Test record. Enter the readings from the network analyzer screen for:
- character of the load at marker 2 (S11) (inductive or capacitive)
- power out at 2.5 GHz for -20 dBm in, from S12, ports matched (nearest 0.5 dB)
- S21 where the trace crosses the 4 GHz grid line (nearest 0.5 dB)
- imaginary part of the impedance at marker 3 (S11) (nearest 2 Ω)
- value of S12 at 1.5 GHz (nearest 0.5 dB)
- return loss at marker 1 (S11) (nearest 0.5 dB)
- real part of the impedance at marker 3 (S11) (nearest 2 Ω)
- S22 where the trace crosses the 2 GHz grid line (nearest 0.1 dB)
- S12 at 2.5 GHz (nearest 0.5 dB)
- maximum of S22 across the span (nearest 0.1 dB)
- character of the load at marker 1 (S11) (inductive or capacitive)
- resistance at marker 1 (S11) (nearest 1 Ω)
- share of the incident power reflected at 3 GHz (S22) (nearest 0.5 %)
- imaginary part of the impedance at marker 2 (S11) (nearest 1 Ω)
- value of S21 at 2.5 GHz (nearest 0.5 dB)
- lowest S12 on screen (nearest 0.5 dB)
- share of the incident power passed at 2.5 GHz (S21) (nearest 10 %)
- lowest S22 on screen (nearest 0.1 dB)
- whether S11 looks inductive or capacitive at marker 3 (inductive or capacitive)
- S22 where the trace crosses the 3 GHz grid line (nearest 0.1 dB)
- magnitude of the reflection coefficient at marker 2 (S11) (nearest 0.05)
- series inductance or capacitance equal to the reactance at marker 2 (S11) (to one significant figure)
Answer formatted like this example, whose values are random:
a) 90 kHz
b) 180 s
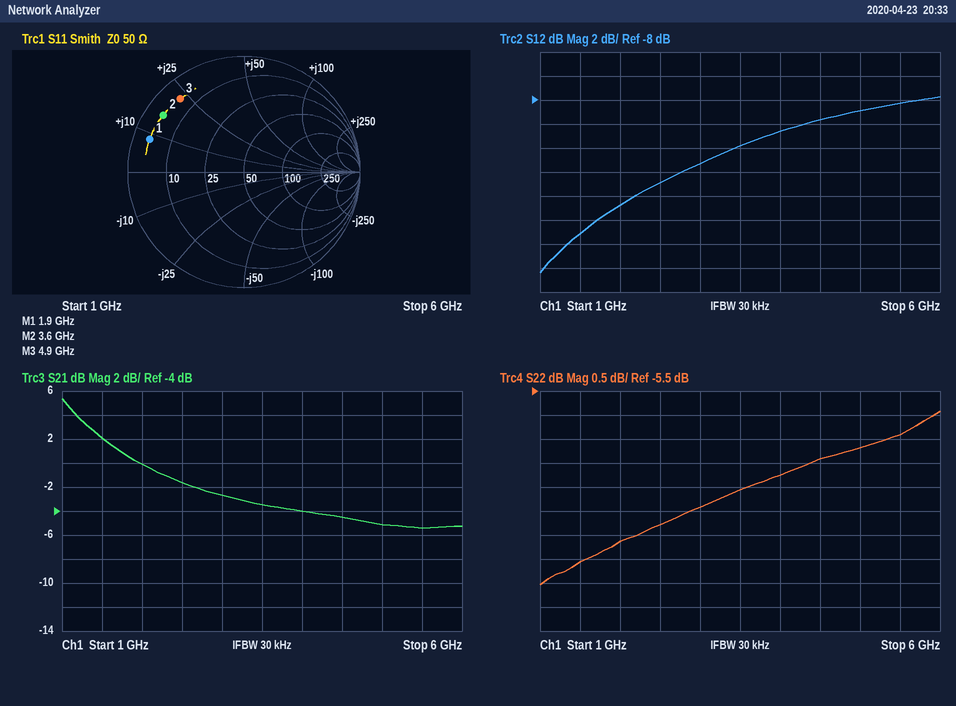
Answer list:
a) inductive
b) -35.0 dBm
c) -4.0 dB
d) +22 Ω
e) -19.0 dB
f) 1.5 dB
g) 6 Ω
h) -8.6 dB
i) -15.0 dB
j) -5.9 dB
k) inductive
l) 4 Ω
m) 16.0 %
n) +16 Ω
o) -1.5 dB
p) -22.5 dB
q) 70 %
r) -9.5 dB
s) inductive
t) -7.9 dB
u) 0.85
v) 700 pH
